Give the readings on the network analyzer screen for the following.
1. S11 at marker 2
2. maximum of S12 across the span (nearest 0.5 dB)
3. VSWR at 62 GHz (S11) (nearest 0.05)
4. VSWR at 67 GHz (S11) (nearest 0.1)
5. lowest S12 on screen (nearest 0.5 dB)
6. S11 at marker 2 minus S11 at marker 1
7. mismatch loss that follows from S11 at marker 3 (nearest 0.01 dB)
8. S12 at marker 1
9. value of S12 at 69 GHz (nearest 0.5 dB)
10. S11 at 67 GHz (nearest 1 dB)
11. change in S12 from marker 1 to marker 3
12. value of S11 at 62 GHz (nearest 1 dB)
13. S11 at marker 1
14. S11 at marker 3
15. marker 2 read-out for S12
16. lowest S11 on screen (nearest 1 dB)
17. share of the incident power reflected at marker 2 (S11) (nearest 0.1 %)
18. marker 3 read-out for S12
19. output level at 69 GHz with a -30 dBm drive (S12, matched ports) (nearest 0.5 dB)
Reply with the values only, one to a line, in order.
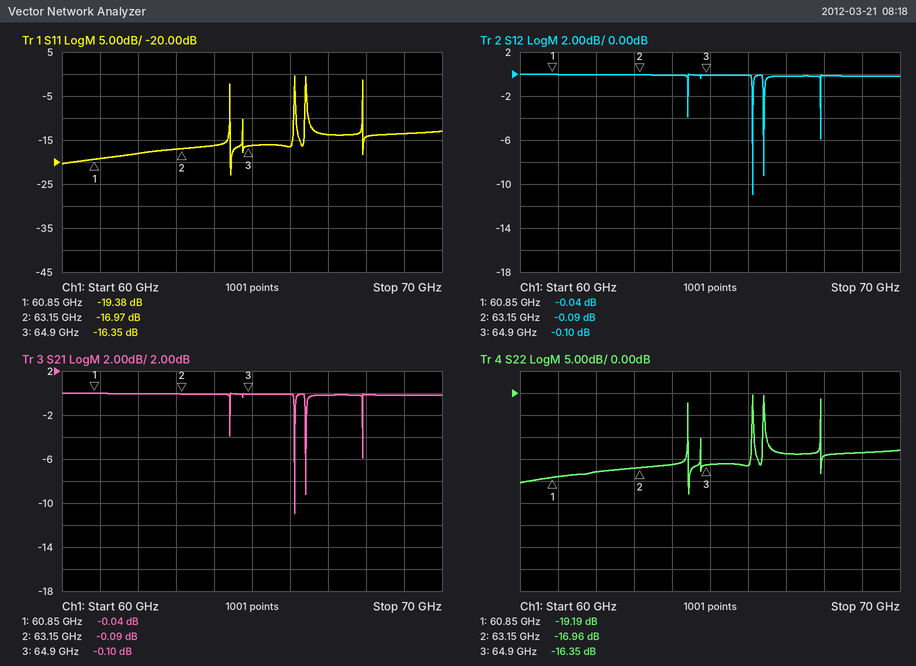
-16.97 dB
0.0 dB
1.30
1.5
-11.0 dB
2.41 dB
0.10 dB
-0.04 dB
0.0 dB
-14 dB
-0.06 dB
-18 dB
-19.38 dB
-16.35 dB
-0.09 dB
-23 dB
2.0 %
-0.10 dB
-30.0 dBm
